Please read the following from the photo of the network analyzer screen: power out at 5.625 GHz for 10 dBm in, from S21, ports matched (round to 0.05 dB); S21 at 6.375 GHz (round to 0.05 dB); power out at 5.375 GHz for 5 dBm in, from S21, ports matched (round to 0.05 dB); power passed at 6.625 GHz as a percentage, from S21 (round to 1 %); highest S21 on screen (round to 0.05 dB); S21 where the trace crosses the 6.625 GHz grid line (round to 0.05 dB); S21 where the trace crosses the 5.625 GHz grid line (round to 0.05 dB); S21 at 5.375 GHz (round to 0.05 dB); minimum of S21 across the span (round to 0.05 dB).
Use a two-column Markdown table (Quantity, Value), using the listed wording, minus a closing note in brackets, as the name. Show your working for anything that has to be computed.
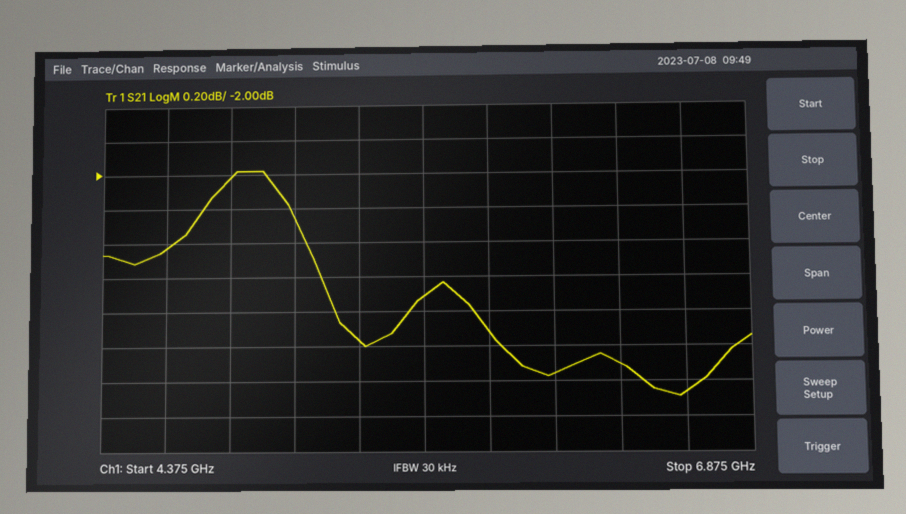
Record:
| Quantity | Value |
|---|---|
| power out at 5.625 GHz for 10 dBm in, from S21, ports matched | 10 dBm + (-2.70 dB) = 7.30 dBm |
| S21 at 6.375 GHz | -3.10 dB |
| power out at 5.375 GHz for 5 dBm in, from S21, ports matched | 5 dBm + (-2.95 dB) = 2.05 dBm |
| power passed at 6.625 GHz as a percentage, from S21 | 10^(-3.25/10) ≈ 47 % |
| highest S21 on screen | -2.00 dB |
| S21 where the trace crosses the 6.625 GHz grid line | -3.25 dB |
| S21 where the trace crosses the 5.625 GHz grid line | -2.70 dB |
| S21 at 5.375 GHz | -2.95 dB |
| minimum of S21 across the span | -3.30 dB |
